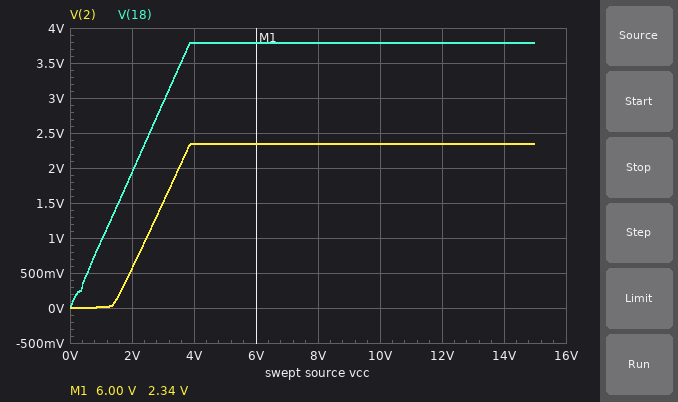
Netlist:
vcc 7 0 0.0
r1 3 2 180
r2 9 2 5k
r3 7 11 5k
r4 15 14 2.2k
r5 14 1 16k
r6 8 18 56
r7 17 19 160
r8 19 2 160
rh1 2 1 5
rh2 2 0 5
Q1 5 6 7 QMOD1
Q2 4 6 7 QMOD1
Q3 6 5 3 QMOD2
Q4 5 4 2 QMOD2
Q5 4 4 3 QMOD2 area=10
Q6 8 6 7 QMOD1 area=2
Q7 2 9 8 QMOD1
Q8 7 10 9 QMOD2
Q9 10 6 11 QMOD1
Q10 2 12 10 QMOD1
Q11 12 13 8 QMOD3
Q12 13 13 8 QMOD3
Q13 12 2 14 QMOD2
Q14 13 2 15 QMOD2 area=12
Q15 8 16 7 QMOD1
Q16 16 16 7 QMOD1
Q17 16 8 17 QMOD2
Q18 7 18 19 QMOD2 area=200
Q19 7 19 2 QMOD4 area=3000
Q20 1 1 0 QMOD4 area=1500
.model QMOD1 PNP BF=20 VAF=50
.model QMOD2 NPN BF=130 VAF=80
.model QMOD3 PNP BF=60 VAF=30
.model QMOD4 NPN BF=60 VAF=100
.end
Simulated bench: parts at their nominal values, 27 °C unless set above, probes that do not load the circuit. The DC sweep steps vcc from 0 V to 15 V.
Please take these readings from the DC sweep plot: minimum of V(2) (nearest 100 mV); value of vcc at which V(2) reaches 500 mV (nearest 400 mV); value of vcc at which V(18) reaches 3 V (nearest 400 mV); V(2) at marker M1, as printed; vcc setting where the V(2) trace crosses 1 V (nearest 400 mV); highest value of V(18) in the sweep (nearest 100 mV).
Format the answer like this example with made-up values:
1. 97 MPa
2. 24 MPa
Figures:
1. 0 V
2. 2.0 V
3. 3.2 V
4. 2.34 V
5. 2.4 V
6. 3.8 V
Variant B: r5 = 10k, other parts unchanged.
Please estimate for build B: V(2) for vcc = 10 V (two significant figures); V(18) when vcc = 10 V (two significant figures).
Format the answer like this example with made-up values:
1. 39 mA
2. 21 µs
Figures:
1. 2.0 V
2. 3.4 V
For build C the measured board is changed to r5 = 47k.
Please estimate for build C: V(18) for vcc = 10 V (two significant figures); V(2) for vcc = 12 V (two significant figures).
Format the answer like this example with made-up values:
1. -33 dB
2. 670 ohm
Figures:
1. 5.6 V
2. 4.2 V
